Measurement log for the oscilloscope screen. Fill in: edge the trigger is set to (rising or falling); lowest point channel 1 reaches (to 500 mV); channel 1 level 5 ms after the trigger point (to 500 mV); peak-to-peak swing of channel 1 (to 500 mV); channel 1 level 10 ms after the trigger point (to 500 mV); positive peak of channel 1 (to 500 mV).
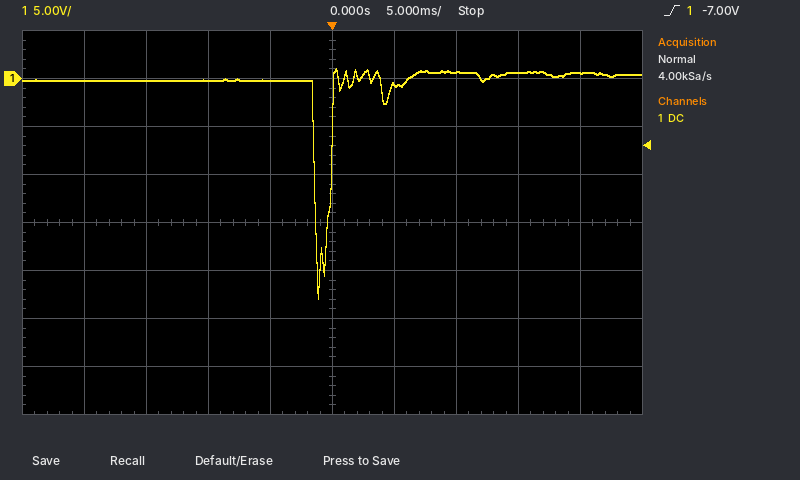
rising
-23.0 V
-500 mV
24.0 V
500 mV
1.0 V
